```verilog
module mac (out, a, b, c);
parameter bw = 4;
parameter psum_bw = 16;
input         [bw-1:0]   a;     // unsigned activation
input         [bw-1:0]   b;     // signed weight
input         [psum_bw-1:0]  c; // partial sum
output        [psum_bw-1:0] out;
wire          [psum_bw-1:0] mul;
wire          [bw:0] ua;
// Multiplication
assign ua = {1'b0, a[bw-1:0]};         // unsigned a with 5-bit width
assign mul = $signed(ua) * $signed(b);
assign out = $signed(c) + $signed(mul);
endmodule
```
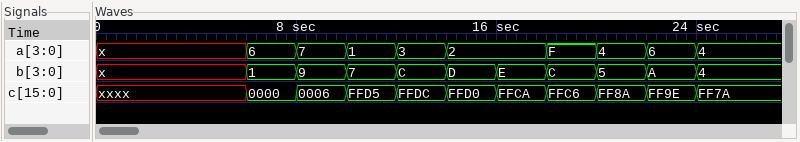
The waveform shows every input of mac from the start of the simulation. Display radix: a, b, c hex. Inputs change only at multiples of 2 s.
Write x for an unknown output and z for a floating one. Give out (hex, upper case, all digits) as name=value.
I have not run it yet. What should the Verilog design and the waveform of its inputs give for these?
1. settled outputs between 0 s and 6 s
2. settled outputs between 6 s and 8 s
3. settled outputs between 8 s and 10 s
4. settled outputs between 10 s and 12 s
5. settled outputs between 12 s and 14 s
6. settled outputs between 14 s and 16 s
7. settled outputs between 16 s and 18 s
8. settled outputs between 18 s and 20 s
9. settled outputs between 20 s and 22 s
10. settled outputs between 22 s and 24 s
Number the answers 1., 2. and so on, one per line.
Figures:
1. out=x
2. out=0006
3. out=FFD5
4. out=FFDC
5. out=FFD0
6. out=FFCA
7. out=FFC6
8. out=FF8A
9. out=FF9E
10. out=FF7A
